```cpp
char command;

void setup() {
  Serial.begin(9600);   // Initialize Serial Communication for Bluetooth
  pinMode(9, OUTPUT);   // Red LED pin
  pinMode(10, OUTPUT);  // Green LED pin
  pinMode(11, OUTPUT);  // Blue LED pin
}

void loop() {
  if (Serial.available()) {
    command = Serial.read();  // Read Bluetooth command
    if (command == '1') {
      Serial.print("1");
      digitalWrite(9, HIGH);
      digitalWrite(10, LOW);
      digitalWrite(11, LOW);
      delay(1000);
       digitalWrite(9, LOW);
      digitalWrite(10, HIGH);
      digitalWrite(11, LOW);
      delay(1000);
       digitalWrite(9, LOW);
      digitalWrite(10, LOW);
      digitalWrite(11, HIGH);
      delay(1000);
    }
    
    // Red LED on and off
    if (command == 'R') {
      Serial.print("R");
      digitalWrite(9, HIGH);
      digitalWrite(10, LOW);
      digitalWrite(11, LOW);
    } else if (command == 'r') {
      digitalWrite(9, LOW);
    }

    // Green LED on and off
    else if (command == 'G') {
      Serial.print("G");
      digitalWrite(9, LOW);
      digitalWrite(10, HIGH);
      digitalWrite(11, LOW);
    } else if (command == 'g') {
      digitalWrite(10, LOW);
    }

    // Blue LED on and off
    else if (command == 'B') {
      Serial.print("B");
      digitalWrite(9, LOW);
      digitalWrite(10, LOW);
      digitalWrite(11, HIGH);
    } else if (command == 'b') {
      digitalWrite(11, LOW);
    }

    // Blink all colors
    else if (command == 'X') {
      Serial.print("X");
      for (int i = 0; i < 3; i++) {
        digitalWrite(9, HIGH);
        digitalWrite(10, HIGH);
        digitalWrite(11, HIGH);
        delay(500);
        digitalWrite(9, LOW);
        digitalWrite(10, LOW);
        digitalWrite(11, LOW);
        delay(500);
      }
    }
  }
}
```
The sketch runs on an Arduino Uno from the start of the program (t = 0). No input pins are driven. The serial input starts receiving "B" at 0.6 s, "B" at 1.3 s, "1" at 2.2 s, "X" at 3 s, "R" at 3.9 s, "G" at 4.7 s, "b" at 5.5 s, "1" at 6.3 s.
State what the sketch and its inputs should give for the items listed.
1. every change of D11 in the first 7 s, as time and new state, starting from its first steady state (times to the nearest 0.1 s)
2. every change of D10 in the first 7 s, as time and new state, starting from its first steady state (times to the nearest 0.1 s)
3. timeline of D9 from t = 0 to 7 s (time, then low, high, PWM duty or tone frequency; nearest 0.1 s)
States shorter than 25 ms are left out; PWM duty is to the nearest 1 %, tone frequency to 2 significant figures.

0 s low; 0.6 s high; 2.2 s low; 4.2 s high; 5.7 s low; 6.2 s high; 6.7 s low
0 s low; 3.2 s high; 4.2 s low; 5.2 s high; 5.7 s low; 6.2 s high; 6.7 s low
0 s low; 2.2 s high; 3.2 s low; 5.2 s high; 5.7 s low; 6.2 s high; 6.7 s low
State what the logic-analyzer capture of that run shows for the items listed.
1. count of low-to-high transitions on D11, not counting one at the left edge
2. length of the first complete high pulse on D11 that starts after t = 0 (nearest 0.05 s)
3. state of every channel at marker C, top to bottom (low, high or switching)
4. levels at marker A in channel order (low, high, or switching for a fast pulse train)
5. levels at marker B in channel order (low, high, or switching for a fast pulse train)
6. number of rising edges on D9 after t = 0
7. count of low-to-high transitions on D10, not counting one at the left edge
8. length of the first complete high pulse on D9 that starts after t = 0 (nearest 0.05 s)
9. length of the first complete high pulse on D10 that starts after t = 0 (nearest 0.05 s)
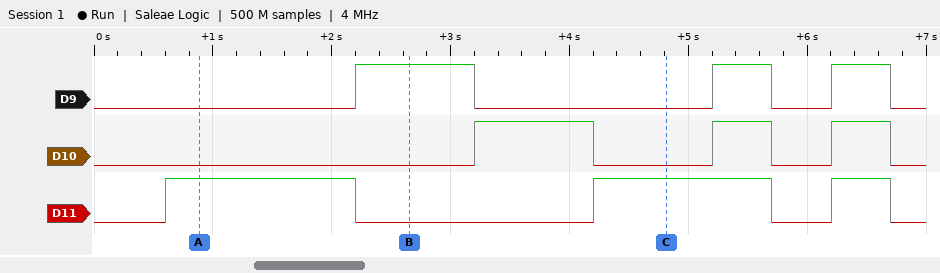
3
1.60 s
D9 low, D10 low, D11 high
D9 low, D10 low, D11 high
D9 high, D10 low, D11 low
3
3
1.00 s
1.00 s
